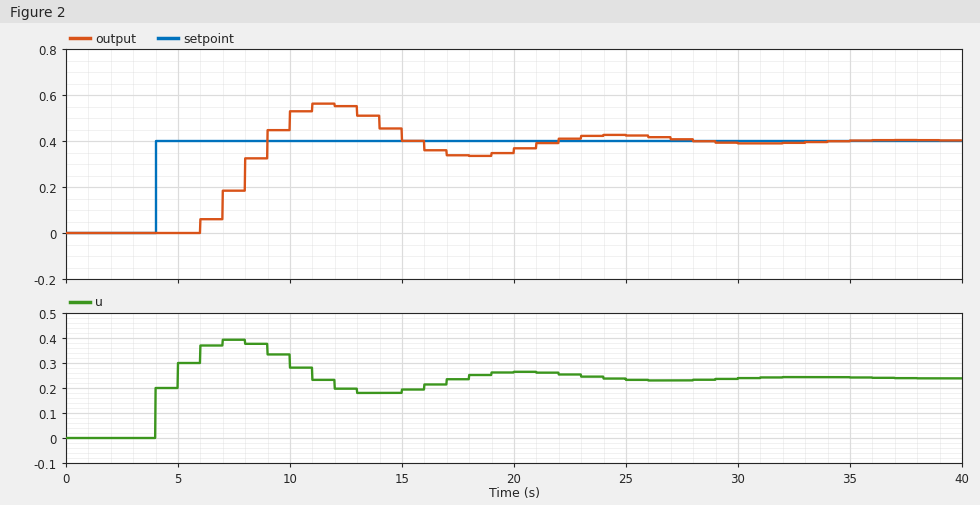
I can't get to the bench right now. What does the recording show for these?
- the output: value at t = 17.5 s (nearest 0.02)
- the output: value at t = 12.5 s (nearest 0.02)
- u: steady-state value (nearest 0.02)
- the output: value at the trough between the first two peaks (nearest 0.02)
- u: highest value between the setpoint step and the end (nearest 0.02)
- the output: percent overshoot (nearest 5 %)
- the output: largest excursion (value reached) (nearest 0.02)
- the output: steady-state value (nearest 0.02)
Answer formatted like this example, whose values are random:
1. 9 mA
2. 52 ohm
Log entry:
1. 0.34
2. 0.56
3. 0.24
4. 0.34
5. 0.40
6. 40 %
7. 0.56
8. 0.40
